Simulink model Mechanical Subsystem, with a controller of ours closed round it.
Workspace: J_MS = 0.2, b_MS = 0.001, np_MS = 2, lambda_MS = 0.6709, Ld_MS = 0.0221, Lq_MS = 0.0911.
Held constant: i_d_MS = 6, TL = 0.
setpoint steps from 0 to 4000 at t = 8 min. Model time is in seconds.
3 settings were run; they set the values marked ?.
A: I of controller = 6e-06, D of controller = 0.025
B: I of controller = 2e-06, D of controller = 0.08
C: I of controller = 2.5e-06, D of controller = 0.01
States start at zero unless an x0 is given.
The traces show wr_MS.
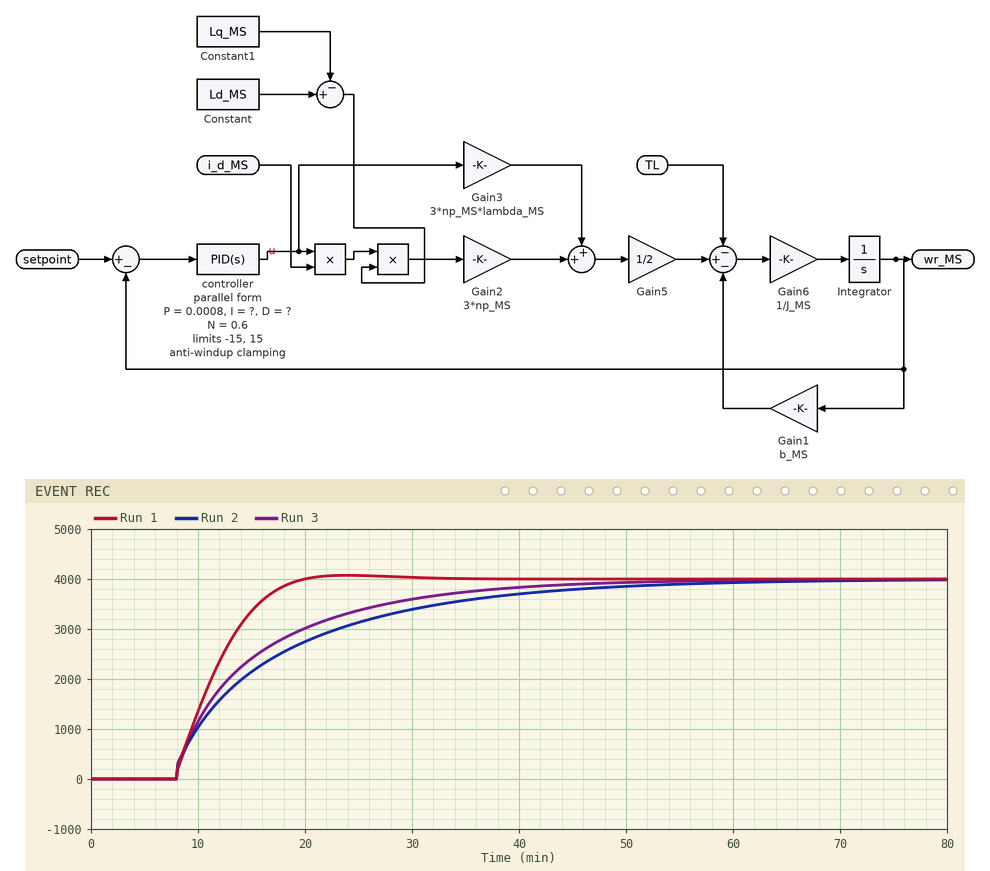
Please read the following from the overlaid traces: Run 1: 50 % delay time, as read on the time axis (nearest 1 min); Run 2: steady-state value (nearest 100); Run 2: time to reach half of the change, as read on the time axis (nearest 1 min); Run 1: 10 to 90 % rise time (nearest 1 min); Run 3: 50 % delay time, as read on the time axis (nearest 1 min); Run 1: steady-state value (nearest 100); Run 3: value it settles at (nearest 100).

11 min
4000
14 min
8 min
13 min
4000
4000
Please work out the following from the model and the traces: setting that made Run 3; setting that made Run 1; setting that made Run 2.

C
A
B
